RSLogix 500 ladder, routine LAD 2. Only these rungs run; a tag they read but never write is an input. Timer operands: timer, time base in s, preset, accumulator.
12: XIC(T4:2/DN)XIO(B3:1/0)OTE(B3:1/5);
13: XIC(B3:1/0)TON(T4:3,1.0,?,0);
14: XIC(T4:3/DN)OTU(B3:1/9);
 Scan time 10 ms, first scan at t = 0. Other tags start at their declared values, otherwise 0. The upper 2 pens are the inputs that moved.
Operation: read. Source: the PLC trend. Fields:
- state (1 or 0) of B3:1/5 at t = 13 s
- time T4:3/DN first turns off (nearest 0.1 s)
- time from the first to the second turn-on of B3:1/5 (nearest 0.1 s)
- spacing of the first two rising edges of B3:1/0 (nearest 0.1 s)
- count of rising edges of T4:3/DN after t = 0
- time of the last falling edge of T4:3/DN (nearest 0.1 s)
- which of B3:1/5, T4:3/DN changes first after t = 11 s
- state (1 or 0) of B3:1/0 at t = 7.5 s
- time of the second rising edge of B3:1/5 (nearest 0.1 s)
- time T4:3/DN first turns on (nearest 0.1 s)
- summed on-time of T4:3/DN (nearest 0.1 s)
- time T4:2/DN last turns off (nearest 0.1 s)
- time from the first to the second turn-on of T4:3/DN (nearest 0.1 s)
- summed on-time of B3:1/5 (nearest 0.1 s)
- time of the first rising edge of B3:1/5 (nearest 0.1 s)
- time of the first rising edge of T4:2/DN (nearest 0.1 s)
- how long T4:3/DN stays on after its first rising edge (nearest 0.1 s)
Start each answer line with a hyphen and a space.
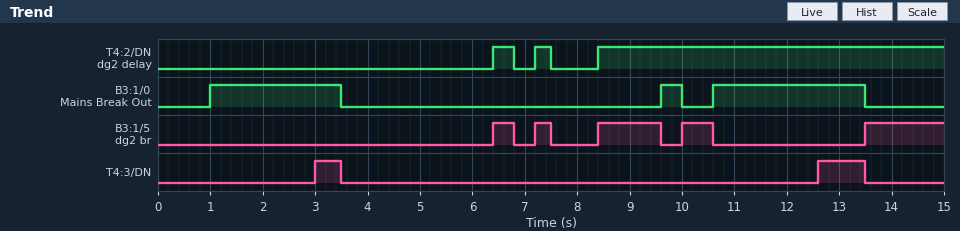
- 0
- 3.5 s
- 0.8 s
- 8.6 s
- 2
- 13.5 s
- T4:3/DN
- 0
- 7.2 s
- 3.0 s
- 1.4 s
- 7.5 s
- 9.6 s
- 4.0 s
- 6.4 s
- 6.4 s
- 0.5 s
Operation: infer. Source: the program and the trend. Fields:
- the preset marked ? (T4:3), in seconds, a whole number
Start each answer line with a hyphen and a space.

- 2 s
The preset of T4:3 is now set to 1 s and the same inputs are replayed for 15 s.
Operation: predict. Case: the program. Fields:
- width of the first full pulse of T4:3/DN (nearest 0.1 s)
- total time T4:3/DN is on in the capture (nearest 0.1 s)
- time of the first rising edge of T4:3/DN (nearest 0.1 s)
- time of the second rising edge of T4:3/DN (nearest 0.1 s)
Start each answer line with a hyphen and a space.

- 1.5 s
- 3.4 s
- 2.0 s
- 11.6 s
